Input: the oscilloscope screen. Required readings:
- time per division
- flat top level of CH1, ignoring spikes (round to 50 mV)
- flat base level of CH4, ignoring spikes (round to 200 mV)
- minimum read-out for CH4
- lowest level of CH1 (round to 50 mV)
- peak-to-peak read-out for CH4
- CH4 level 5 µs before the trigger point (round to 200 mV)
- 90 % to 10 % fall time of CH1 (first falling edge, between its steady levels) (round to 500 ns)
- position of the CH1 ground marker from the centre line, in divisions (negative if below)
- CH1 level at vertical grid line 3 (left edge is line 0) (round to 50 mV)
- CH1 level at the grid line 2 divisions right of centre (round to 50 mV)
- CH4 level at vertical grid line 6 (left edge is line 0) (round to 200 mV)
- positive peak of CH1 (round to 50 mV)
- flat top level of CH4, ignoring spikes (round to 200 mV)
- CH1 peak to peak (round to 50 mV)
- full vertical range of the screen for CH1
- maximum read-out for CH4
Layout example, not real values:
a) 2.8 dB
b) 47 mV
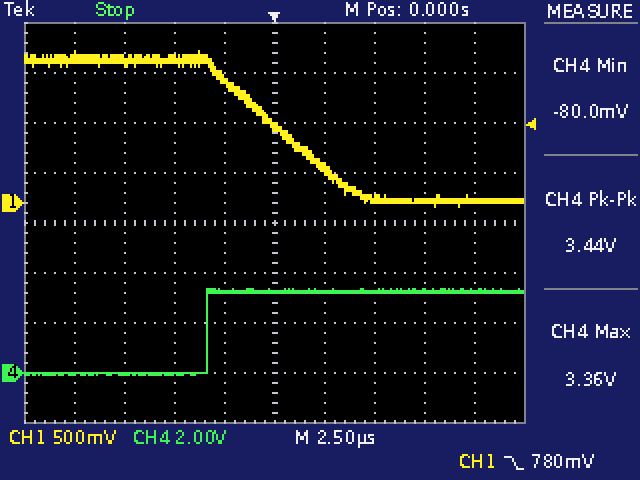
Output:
a) 2.5 µs
b) 1.45 V
c) 0.0 V
d) -80.0 mV
e) -50 mV
f) 3.44 V
g) 0.0 V
h) 6.5 µs
i) +0.4 div
j) 1.45 V
k) 50 mV
l) 3.2 V
m) 1.50 V
n) 3.2 V
o) 1.55 V
p) 4 V
q) 3.36 V
